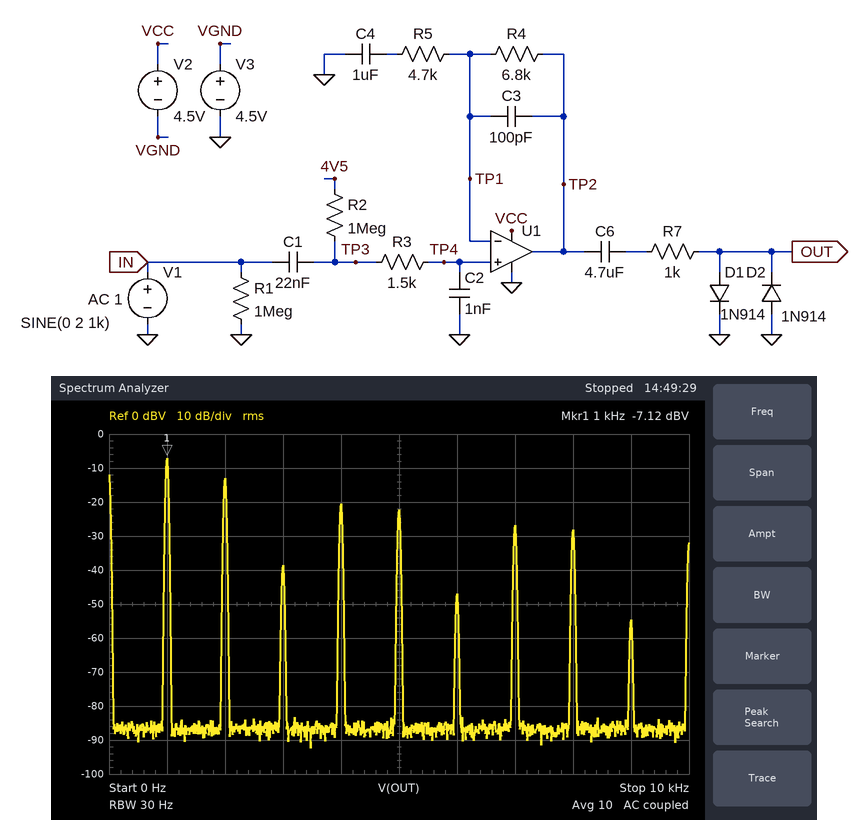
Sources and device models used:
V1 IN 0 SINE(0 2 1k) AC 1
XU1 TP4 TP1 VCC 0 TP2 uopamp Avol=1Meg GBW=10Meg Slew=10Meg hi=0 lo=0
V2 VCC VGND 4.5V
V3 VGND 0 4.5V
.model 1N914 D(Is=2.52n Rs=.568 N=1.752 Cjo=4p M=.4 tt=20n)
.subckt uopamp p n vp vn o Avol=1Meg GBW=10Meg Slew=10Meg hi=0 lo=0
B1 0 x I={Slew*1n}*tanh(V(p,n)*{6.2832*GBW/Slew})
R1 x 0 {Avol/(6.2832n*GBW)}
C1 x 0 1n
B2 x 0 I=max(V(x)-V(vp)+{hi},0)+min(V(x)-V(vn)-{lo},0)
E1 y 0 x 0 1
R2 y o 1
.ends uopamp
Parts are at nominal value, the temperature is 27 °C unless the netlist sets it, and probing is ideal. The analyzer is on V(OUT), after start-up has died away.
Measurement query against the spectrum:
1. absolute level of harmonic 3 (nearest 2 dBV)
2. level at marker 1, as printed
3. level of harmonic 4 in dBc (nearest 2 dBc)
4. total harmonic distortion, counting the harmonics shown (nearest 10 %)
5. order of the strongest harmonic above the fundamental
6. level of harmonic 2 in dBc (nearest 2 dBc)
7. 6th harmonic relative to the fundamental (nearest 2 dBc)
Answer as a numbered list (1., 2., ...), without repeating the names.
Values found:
1. -38 dBV
2. -7.12 dBV
3. -14 dBc
4. 60 %
5. 2
6. -6 dBc
7. -40 dBc
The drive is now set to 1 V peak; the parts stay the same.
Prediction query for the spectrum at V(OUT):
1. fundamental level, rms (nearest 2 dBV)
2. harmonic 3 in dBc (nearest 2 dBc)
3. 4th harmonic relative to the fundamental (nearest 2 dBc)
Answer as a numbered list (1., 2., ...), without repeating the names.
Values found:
1. -8 dBV
2. -22 dBc
3. -16 dBc
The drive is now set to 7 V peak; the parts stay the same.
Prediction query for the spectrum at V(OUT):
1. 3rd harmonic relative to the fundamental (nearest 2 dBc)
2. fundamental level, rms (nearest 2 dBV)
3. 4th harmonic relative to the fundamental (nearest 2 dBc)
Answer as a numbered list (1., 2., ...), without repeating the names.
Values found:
1. -24 dBc
2. -6 dBV
3. -12 dBc
